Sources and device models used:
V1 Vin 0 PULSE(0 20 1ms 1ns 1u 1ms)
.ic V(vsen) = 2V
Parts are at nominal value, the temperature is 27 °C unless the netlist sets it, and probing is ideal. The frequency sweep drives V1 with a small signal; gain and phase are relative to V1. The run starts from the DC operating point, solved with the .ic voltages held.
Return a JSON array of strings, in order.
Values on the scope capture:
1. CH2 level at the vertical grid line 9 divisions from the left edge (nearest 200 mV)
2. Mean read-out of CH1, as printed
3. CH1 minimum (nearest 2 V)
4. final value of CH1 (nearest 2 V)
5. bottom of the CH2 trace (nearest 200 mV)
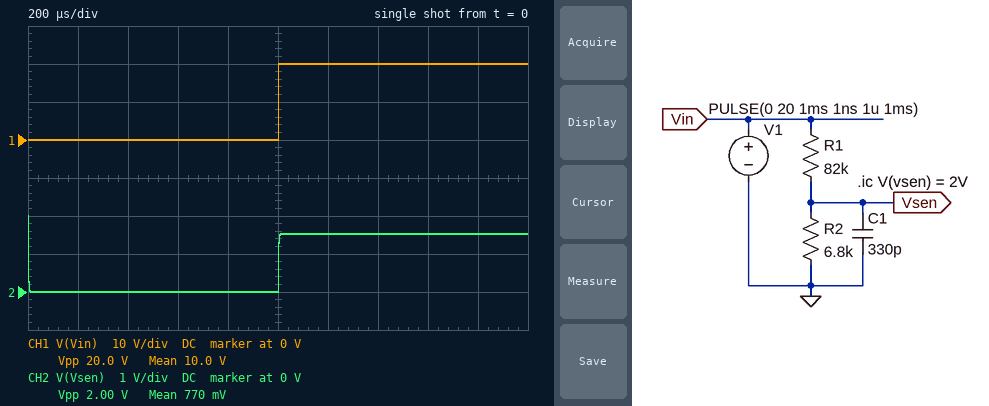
["1.6 V", "10.0 V", "0 V", "20 V", "0 V"]
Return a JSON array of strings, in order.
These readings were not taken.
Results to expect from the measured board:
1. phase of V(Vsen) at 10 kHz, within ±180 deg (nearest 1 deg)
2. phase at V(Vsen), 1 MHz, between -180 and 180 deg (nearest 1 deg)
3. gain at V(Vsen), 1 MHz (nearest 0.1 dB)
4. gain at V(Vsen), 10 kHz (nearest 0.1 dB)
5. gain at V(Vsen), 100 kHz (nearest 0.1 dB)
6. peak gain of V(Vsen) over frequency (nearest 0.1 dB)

["-7 deg", "-86 deg", "-44.6 dB", "-22.4 dB", "-26.6 dB", "-22.3 dB"]
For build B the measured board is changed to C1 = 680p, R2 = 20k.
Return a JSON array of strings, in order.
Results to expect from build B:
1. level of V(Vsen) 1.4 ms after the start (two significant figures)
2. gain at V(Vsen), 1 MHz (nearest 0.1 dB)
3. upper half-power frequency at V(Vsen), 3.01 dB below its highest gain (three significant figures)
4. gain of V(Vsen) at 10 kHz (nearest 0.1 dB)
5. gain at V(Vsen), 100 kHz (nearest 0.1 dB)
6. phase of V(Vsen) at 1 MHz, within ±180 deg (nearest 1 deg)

["3.9 V", "-50.9 dB", "14.6 kHz", "-15.8 dB", "-31.0 dB", "-89 deg"]
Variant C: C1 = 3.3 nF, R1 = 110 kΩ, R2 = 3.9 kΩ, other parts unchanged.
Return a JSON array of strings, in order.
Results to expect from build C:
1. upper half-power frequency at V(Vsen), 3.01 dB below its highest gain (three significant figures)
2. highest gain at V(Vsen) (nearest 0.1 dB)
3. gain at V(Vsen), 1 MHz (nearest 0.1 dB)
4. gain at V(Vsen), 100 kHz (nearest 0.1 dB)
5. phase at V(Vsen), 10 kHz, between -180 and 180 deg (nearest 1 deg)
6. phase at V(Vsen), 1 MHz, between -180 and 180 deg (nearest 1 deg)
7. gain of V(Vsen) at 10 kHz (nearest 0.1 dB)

["12.8 kHz", "-29.3 dB", "-67.2 dB", "-47.2 dB", "-38 deg", "-89 deg", "-31.4 dB"]
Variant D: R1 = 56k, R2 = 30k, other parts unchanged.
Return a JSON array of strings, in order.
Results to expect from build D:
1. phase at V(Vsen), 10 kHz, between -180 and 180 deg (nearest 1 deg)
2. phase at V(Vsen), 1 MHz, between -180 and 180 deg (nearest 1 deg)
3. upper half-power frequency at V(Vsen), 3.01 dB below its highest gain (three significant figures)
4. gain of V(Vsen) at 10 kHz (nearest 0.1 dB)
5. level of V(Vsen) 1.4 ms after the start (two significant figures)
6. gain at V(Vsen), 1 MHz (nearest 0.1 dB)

["-22 deg", "-89 deg", "24.7 kHz", "-9.8 dB", "7.0 V", "-41.3 dB"]
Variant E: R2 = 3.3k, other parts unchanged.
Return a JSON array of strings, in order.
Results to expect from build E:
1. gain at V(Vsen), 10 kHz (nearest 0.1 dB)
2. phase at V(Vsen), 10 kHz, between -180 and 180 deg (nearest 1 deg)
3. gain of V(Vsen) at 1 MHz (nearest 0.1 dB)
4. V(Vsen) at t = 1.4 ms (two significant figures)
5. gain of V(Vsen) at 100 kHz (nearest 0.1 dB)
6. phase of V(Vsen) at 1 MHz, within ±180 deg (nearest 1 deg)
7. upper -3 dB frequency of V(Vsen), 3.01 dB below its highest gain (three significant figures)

["-28.3 dB", "-4 deg", "-44.7 dB", "770 mV", "-29.8 dB", "-81 deg", "152 kHz"]
